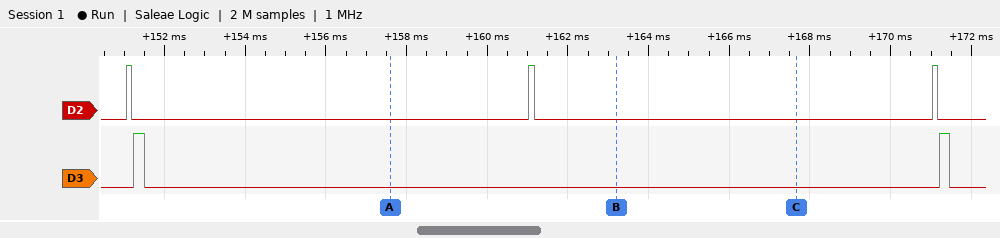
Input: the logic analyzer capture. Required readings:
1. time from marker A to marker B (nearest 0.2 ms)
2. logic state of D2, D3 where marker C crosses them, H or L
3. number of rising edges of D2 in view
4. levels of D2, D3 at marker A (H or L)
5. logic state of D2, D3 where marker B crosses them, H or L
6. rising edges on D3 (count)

5.6 ms
D2=L, D3=L
3
D2=L, D3=L
D2=L, D3=L
2
